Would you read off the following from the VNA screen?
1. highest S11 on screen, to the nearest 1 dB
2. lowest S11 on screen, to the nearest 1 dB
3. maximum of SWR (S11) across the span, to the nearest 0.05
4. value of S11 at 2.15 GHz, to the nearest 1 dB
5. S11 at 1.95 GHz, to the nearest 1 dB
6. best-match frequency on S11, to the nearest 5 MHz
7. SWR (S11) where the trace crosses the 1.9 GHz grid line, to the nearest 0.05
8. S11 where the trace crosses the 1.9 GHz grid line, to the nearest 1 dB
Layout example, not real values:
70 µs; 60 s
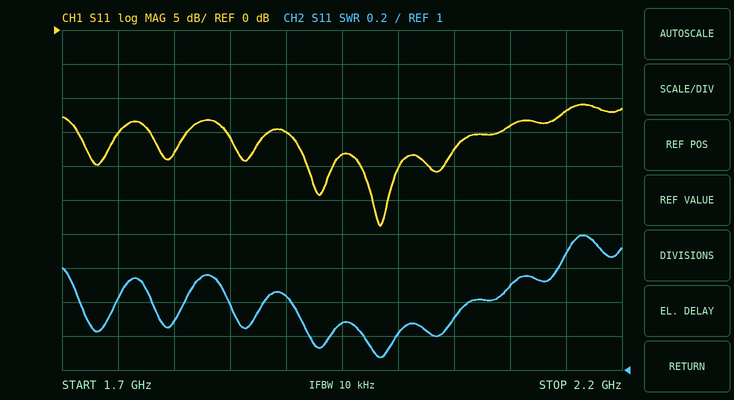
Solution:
-11 dB; -29 dB; 1.80; -12 dB; -18 dB; 1.985 GHz; 1.45; -15 dB
